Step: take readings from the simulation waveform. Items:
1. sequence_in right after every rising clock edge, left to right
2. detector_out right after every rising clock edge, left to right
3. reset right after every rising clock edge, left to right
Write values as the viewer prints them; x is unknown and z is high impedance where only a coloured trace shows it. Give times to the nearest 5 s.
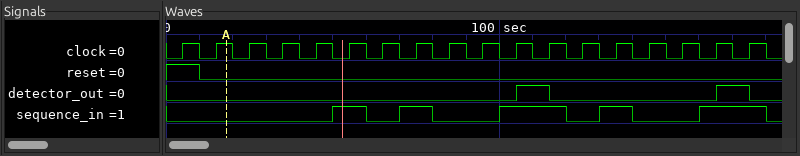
0 0 0 0 0 1 0 1 0 0 1 1 0 1 0 0 1 1
0 0 0 0 0 0 0 0 0 0 1 0 0 0 0 0 1 0
1 0 0 0 0 0 0 0 0 0 0 0 0 0 0 0 0 0
